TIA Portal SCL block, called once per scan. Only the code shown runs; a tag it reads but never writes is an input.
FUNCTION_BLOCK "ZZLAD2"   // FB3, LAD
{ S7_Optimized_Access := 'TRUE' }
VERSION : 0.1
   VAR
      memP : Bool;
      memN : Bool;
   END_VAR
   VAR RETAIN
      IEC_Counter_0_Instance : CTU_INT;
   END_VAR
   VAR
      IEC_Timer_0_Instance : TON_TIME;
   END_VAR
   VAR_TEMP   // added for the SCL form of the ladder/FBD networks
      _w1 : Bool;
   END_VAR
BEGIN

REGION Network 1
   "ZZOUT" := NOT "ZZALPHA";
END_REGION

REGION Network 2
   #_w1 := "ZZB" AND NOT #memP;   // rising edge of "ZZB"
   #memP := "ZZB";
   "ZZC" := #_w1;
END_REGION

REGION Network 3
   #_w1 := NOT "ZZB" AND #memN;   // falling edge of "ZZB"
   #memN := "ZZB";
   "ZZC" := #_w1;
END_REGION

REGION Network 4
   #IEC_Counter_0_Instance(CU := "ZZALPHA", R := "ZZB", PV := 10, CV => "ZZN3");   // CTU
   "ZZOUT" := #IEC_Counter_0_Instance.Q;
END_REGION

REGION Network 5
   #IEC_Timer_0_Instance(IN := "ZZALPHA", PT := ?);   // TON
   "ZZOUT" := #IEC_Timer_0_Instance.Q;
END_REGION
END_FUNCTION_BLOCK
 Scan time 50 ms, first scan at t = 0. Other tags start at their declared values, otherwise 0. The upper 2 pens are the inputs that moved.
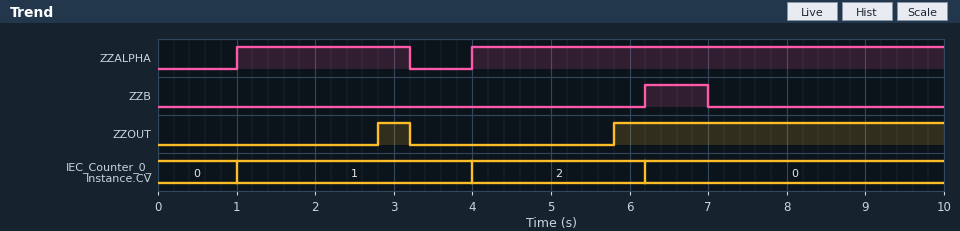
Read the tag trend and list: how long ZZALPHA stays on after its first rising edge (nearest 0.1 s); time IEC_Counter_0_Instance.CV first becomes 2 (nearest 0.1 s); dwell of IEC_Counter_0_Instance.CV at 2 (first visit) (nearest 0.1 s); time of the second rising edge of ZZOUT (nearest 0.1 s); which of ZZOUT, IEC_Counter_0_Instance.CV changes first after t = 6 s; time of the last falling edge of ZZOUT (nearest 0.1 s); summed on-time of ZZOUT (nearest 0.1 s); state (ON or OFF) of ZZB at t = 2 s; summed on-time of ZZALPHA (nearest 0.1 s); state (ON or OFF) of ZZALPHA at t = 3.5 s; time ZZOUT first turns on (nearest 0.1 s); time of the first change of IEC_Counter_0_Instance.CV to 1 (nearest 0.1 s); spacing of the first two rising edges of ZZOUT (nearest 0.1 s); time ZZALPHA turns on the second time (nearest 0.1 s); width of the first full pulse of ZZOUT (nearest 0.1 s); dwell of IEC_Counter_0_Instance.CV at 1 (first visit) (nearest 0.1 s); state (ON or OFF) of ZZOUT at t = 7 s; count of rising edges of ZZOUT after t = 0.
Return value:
2.2 s
4.0 s
2.2 s
5.8 s
IEC_Counter_0_Instance.CV
3.2 s
4.6 s
OFF
8.2 s
OFF
2.8 s
1.0 s
3.0 s
4.0 s
0.4 s
3.0 s
ON
2
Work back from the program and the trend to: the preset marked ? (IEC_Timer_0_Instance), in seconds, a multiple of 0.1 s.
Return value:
1.8 s
